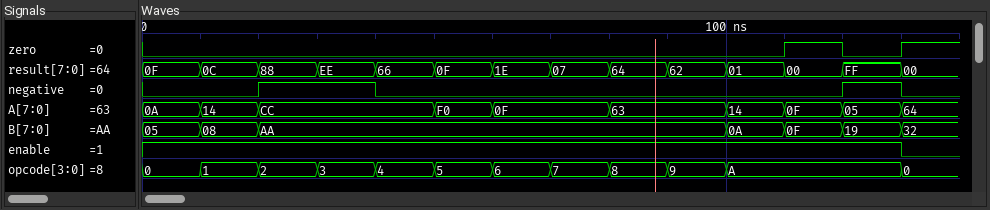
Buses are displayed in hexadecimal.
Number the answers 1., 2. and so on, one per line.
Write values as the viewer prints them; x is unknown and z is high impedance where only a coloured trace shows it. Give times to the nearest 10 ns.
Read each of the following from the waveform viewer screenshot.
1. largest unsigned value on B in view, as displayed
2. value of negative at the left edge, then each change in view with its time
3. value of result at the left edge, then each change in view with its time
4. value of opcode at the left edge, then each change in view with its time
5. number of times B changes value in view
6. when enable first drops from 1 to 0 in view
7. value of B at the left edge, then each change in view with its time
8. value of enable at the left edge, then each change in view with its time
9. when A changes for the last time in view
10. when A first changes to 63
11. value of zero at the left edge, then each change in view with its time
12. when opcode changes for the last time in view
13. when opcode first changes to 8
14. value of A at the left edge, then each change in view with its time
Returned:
1. AA
2. 0, 1 at 20 ns, 0 at 40 ns, 1 at 120 ns, 0 at 130 ns
3. 0F, 0C at 10 ns, 88 at 20 ns, EE at 30 ns, 66 at 40 ns, 0F at 50 ns, 1E at 60 ns, 07 at 70 ns, 64 at 80 ns, 62 at 90 ns, 01 at 100 ns, 00 at 110 ns, FF at 120 ns, 00 at 130 ns
4. 0, 1 at 10 ns, 2 at 20 ns, 3 at 30 ns, 4 at 40 ns, 5 at 50 ns, 6 at 60 ns, 7 at 70 ns, 8 at 80 ns, 9 at 90 ns, A at 100 ns, 0 at 130 ns
5. 6
6. 130 ns
7. 05, 08 at 10 ns, AA at 20 ns, 0A at 100 ns, 0F at 110 ns, 19 at 120 ns, 32 at 130 ns
8. 1, 0 at 130 ns
9. 130 ns
10. 80 ns
11. 0, 1 at 110 ns, 0 at 120 ns, 1 at 130 ns
12. 130 ns
13. 80 ns
14. 0A, 14 at 10 ns, CC at 20 ns, F0 at 50 ns, 0F at 60 ns, 63 at 80 ns, 14 at 100 ns, 0F at 110 ns, 05 at 120 ns, 64 at 130 ns
